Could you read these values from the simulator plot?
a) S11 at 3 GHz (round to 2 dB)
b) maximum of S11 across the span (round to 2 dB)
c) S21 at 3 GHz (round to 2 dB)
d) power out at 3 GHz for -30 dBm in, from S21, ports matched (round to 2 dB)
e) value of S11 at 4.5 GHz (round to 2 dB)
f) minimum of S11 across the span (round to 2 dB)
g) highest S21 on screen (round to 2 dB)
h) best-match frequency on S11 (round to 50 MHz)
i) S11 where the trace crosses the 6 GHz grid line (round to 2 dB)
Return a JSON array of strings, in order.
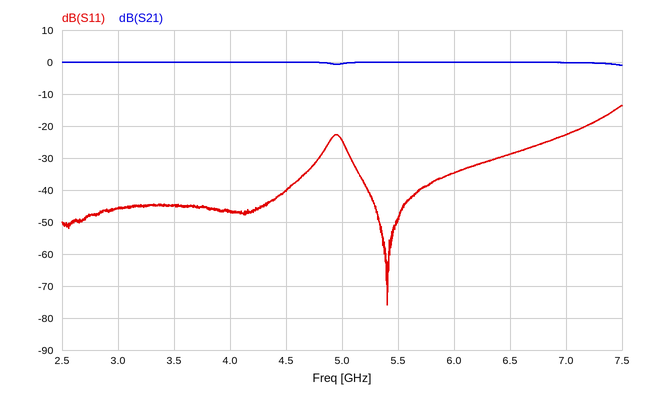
["-46 dB", "-14 dB", "0 dB", "-30 dBm", "-40 dB", "-76 dB", "0 dB", "5.40 GHz", "-34 dB"]
